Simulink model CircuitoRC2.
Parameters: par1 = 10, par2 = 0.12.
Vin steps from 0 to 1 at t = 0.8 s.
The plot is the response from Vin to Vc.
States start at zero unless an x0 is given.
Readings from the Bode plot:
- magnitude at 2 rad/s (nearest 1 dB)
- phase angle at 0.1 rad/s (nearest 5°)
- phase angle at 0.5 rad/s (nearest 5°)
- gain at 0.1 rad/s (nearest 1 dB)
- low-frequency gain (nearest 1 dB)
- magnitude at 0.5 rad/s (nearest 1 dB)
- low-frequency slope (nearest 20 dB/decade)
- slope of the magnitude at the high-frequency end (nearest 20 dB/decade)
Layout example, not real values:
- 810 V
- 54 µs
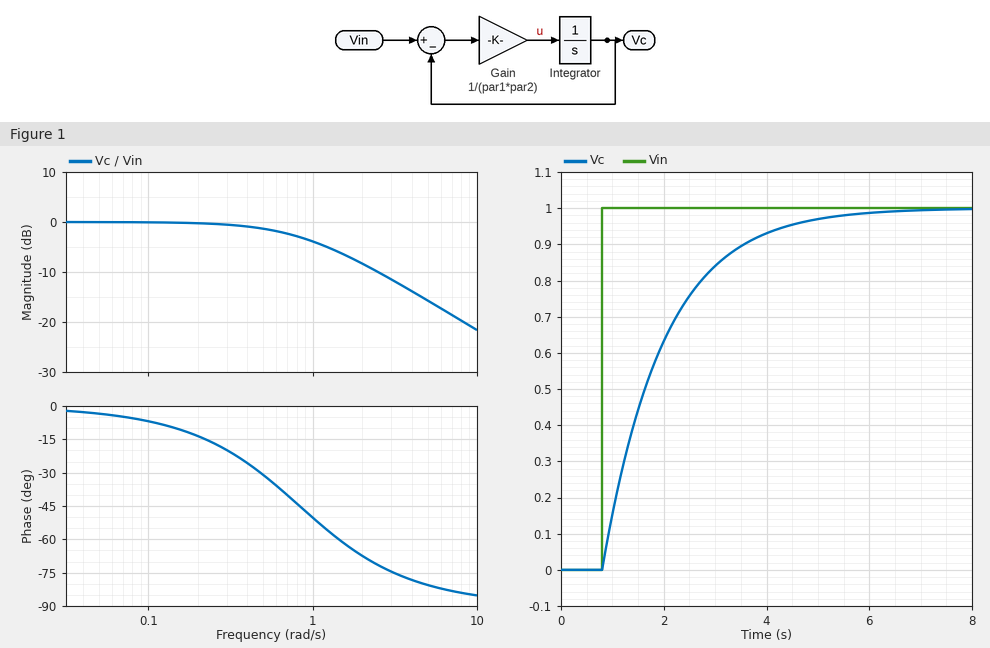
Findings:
- -8 dB
- -5°
- -30°
- 0 dB
- 0 dB
- -1 dB
- 0 dB/decade
- -20 dB/decade
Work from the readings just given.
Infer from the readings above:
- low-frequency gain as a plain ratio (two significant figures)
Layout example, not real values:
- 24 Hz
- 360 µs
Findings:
- 1.0
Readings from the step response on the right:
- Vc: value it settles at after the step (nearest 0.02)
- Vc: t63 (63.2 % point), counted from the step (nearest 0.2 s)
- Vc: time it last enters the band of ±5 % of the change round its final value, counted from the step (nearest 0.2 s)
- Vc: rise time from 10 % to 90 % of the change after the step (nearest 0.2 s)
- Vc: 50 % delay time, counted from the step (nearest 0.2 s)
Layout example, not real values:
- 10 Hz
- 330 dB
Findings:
- 1.00
- 1.2 s
- 3.6 s
- 2.6 s
- 0.8 s
